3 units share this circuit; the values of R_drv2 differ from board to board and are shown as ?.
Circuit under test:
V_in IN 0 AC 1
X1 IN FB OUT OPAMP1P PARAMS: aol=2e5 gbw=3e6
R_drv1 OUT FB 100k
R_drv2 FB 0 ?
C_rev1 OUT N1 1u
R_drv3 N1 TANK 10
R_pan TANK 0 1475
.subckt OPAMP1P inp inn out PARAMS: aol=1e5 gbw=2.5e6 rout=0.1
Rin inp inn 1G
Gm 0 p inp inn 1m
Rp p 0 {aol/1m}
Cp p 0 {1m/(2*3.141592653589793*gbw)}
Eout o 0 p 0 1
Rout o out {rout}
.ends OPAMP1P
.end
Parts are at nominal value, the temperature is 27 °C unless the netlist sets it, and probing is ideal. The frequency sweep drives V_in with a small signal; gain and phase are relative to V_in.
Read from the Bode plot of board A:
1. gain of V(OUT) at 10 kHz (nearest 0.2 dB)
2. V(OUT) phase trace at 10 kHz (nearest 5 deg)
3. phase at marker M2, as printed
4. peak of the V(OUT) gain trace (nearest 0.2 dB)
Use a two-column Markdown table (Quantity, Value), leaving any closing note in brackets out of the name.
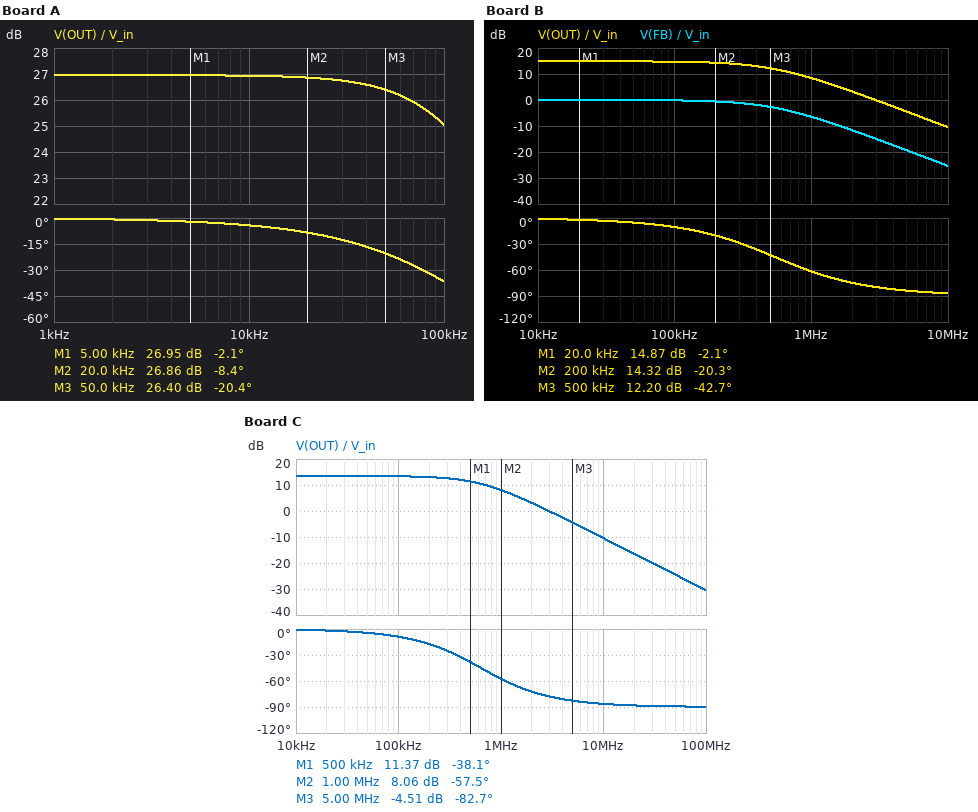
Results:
| Quantity | Value |
|---|---|
| gain of V(OUT) at 10 kHz | 27.0 dB |
| V(OUT) phase trace at 10 kHz | -5 deg |
| phase at marker M2, as printed | -8.4 deg |
| peak of the V(OUT) gain trace | 27.0 dB |
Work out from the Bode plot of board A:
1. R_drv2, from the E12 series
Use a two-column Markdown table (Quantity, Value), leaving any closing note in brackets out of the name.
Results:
| Quantity | Value |
|---|---|
| R_drv2, from the E12 series | 4.7 kΩ |
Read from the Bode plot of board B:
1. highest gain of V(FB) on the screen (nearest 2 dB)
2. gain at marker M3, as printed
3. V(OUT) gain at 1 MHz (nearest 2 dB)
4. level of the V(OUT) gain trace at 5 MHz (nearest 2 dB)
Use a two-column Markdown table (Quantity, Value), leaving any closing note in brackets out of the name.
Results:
| Quantity | Value |
|---|---|
| highest gain of V(FB) on the screen | 0 dB |
| gain at marker M3, as printed | 12.20 dB |
| V(OUT) gain at 1 MHz | 8 dB |
| level of the V(OUT) gain trace at 5 MHz | -4 dB |
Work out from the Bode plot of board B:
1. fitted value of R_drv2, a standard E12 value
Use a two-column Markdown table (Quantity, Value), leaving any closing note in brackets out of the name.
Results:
| Quantity | Value |
|---|---|
| fitted value of R_drv2, a standard E12 value | 22 kΩ |
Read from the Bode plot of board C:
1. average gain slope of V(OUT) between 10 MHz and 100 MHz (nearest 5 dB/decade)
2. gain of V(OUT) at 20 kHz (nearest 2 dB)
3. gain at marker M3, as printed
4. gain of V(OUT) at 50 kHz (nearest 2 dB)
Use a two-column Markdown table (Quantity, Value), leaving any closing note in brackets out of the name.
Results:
| Quantity | Value |
|---|---|
| average gain slope of V(OUT) between 10 MHz and 100 MHz | -20 dB/decade |
| gain of V(OUT) at 20 kHz | 14 dB |
| gain at marker M3, as printed | -4.51 dB |
| gain of V(OUT) at 50 kHz | 14 dB |
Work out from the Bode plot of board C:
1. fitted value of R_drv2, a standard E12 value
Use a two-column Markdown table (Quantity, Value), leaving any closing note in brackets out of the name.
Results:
| Quantity | Value |
|---|---|
| fitted value of R_drv2, a standard E12 value | 27 kΩ |
